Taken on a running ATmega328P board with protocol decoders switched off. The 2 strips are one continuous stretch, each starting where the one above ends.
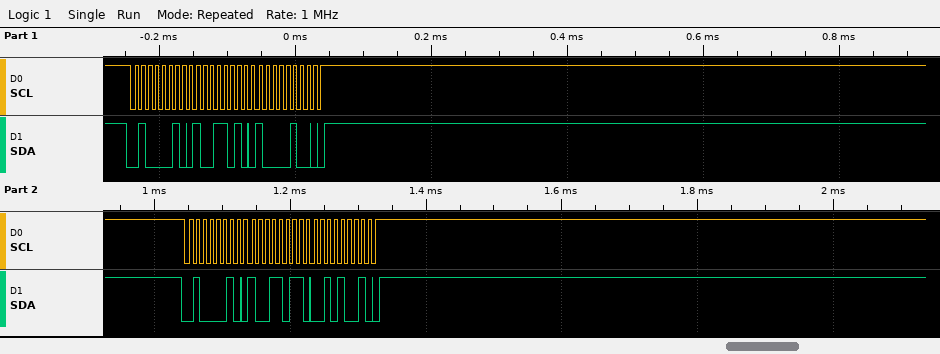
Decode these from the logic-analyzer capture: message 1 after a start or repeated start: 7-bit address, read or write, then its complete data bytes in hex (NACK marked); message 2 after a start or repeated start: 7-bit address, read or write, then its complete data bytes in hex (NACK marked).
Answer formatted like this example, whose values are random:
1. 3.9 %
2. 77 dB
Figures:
1. 0x21 write: 9A 84
2. 0x21 write: 9B 29
